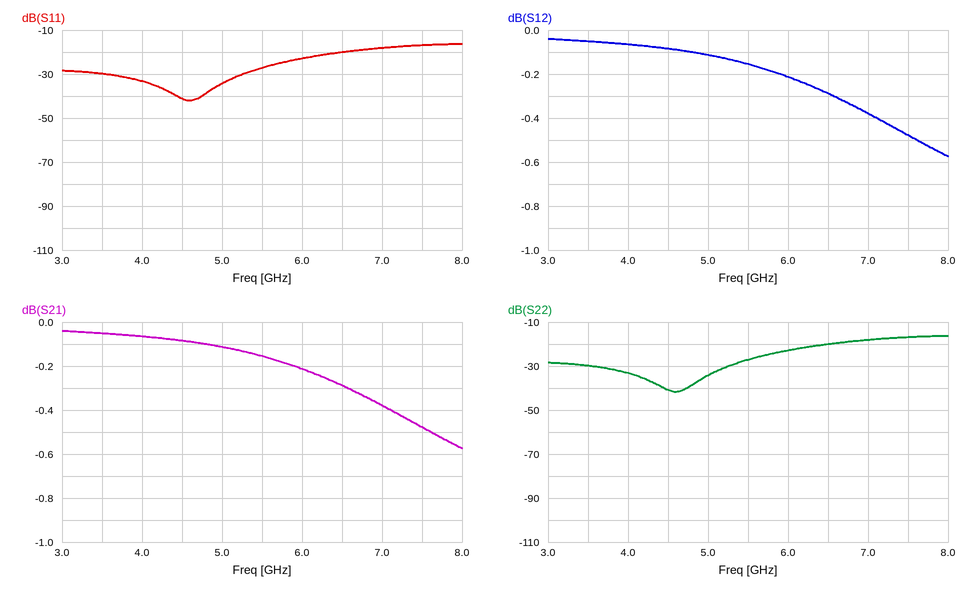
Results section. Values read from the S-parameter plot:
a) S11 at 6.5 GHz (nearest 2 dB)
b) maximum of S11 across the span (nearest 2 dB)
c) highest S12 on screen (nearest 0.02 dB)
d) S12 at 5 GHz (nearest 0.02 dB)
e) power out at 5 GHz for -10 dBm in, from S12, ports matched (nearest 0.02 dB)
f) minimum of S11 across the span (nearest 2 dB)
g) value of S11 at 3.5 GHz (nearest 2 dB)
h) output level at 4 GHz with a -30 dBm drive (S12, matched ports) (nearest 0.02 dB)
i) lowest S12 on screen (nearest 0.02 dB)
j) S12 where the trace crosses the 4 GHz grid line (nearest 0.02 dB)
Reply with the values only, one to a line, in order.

-20 dB
-16 dB
-0.04 dB
-0.12 dB
-10.12 dBm
-42 dB
-30 dB
-30.06 dBm
-0.58 dB
-0.06 dB
